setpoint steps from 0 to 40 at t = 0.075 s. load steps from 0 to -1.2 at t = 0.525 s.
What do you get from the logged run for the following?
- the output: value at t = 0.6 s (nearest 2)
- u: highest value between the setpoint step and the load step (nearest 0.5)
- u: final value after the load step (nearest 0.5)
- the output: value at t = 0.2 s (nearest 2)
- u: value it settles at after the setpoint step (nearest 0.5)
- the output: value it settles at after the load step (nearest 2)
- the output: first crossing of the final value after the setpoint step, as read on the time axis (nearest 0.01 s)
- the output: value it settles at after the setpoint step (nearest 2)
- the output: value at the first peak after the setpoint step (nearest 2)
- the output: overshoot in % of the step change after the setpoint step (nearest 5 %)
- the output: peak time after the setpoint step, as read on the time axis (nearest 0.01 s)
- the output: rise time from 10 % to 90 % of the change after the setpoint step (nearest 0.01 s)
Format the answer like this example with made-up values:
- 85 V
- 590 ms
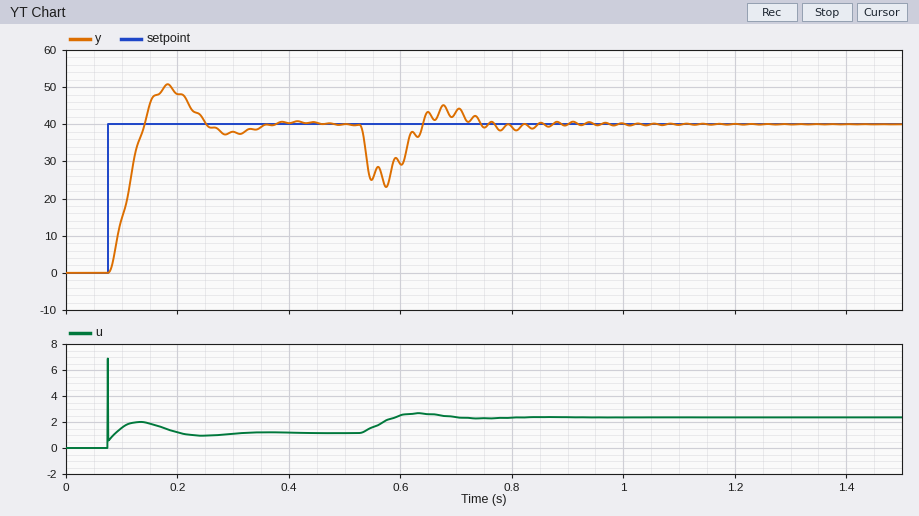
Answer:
- 30
- 7.0
- 2.5
- 48
- 1.0
- 40
- 0.14 s
- 40
- 50
- 25 %
- 0.18 s
- 0.05 s
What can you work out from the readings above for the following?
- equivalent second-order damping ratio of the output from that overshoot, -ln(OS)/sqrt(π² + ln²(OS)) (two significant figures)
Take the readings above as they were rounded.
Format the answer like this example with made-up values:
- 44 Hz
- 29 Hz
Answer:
- 0.40
